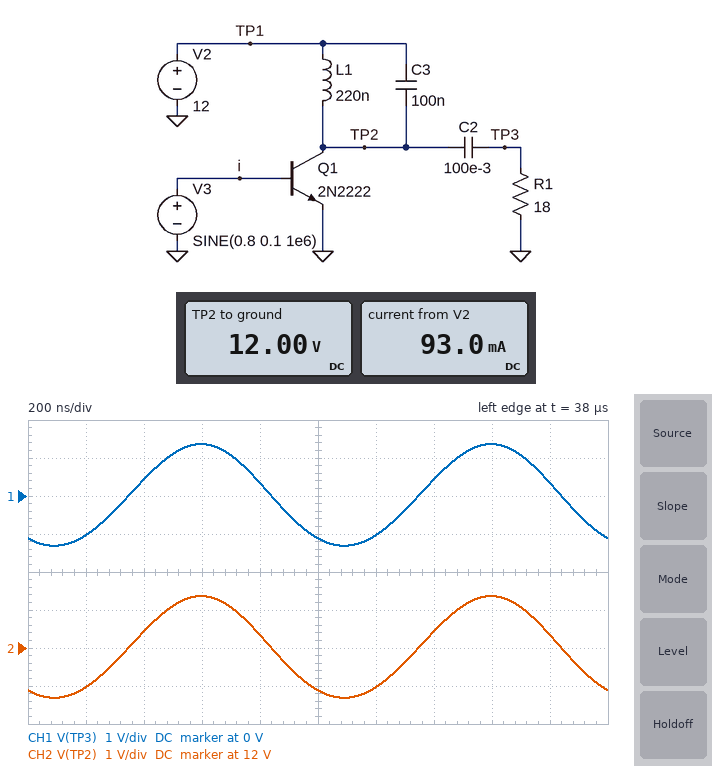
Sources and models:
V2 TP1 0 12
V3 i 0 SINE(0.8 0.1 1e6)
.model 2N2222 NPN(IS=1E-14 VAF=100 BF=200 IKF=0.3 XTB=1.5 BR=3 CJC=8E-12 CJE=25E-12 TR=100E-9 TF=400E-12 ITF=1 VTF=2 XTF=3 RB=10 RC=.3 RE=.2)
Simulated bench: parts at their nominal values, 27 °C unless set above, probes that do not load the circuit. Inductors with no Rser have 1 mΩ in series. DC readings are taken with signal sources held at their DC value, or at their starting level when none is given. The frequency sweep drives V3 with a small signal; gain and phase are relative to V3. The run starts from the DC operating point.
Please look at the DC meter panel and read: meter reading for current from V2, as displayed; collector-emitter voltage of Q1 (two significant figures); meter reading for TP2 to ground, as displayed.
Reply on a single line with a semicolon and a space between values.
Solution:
93.0 mA; 12 V; 12.00 V
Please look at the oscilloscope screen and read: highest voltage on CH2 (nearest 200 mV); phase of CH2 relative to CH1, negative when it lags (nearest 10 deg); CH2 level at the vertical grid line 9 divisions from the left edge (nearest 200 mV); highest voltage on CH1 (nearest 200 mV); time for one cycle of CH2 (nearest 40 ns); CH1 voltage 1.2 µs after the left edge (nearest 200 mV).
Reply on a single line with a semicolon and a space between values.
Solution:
13.4 V; 0 deg; 12.4 V; 1.4 V; 1.00 µs; -1.0 V
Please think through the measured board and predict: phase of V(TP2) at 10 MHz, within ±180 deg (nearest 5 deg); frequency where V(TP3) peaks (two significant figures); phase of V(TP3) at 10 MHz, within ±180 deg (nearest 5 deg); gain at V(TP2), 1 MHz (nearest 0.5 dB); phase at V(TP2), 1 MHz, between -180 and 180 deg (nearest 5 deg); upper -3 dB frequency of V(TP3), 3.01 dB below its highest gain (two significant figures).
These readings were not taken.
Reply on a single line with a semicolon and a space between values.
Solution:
65 deg; 1.1 MHz; 65 deg; 23.5 dB; -125 deg; 1.1 MHz
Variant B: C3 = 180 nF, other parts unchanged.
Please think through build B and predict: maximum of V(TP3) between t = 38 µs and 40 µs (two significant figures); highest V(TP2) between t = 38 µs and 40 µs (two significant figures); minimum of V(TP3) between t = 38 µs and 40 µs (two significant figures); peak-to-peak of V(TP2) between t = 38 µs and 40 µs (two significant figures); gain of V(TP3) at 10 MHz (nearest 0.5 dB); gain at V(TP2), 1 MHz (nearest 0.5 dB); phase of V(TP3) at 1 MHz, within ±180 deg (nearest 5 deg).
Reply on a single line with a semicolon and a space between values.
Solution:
360 mV; 12 V; -370 mV; 720 mV; -17.5 dB; 12.0 dB; 95 deg
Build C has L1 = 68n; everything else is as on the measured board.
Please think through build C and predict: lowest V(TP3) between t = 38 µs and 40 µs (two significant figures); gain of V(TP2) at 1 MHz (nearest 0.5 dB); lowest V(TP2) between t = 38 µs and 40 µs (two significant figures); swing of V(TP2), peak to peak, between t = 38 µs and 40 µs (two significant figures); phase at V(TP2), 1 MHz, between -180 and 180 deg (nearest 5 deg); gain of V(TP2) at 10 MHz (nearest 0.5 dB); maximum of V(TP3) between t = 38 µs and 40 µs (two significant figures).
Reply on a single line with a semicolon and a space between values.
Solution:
-320 mV; -0.5 dB; 12 V; 670 mV; -95 deg; -12.0 dB; 350 mV
